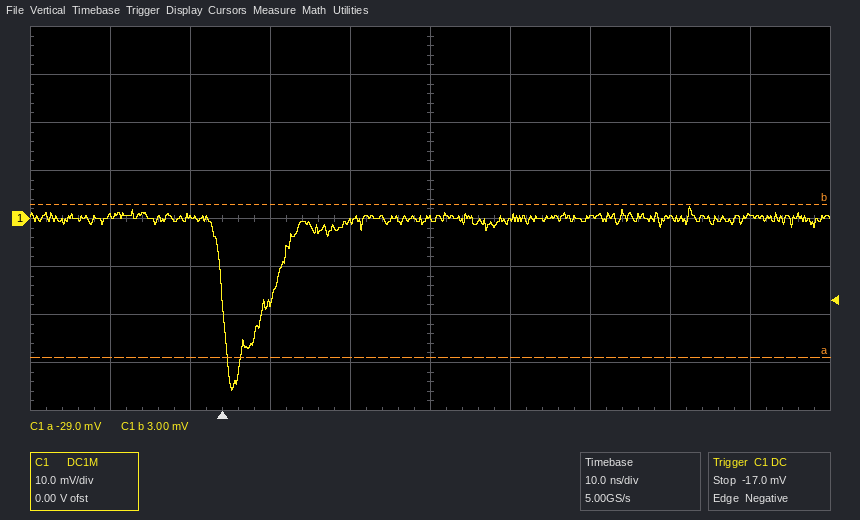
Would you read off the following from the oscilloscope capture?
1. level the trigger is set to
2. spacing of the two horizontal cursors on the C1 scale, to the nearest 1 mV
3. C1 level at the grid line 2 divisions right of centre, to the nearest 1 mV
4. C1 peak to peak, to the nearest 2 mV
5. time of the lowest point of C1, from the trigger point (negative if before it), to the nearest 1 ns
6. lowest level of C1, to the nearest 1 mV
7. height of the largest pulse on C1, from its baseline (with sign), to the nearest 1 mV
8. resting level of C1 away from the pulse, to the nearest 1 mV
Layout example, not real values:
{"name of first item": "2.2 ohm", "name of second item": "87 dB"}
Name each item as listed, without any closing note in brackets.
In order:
{"level the trigger is set to": "-17.0 mV", "spacing of the two horizontal cursors on the C1 scale, to the nearest 1 mV": "32 mV", "C1 level at the grid line 2 divisions right of centre, to the nearest 1 mV": "0 mV", "C1 peak to peak, to the nearest 2 mV": "38 mV", "time of the lowest point of C1, from the trigger point (negative if before it), to the nearest 1 ns": "+1 ns", "lowest level of C1, to the nearest 1 mV": "-36 mV", "height of the largest pulse on C1, from its baseline (with sign), to the nearest 1 mV": "-36 mV", "resting level of C1 away from the pulse, to the nearest 1 mV": "0 mV"}
